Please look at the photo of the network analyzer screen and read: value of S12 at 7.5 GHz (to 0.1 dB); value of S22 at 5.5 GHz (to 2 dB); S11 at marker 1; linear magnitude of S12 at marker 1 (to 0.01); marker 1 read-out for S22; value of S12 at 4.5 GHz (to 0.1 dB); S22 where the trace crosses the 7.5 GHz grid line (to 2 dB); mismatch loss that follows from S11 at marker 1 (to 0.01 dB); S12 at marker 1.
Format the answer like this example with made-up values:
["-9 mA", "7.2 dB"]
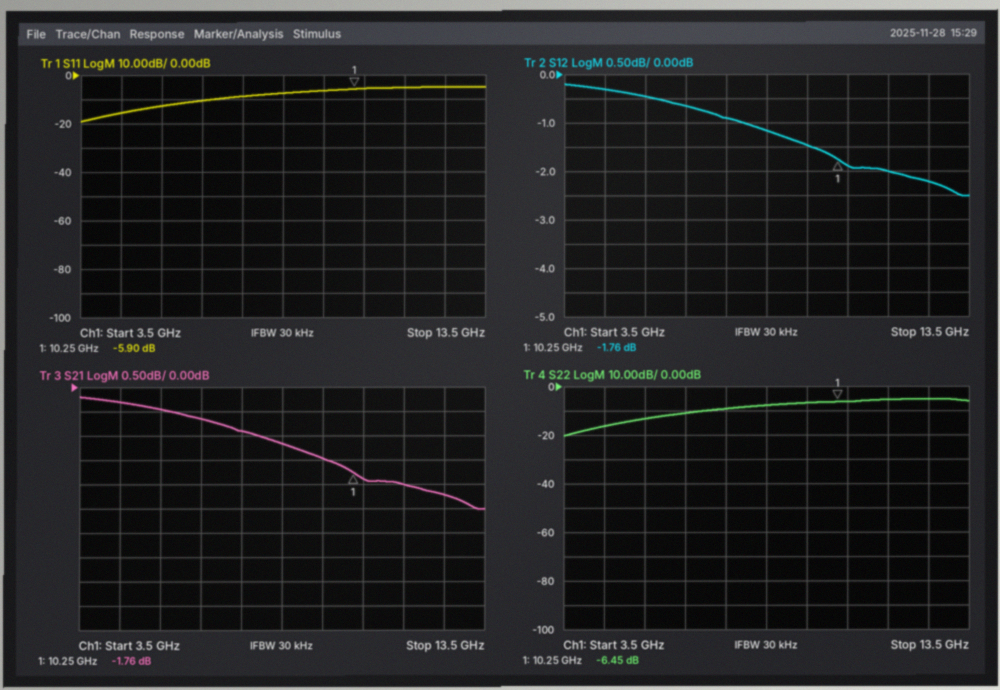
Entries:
["-0.9 dB", "-14 dB", "-5.90 dB", "0.82", "-6.45 dB", "-0.3 dB", "-10 dB", "1.29 dB", "-1.76 dB"]
